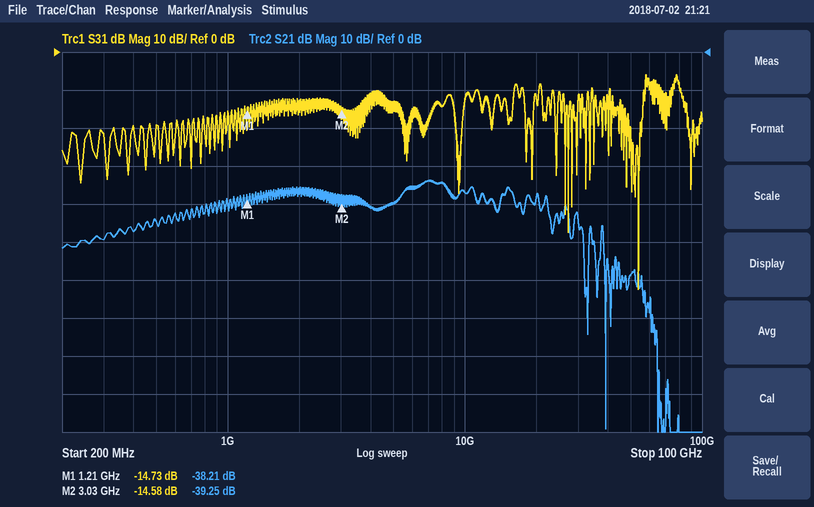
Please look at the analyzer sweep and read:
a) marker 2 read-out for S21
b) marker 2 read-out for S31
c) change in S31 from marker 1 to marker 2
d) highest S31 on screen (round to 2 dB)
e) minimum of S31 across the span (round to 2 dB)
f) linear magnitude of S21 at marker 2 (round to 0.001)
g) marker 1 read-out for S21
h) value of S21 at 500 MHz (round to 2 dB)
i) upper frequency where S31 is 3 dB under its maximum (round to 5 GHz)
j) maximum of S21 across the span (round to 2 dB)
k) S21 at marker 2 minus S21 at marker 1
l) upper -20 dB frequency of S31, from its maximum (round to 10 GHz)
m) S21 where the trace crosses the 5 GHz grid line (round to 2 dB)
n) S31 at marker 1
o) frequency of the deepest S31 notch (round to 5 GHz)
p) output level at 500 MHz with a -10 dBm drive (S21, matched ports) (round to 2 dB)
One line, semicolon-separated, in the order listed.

-39.25 dB; -14.58 dB; 0.15 dB; -6 dB; -62 dB; 0.011; -38.21 dB; -44 dB; 80 GHz; -34 dB; -1.04 dB; 90 GHz; -40 dB; -14.73 dB; 55 GHz; -54 dBm
